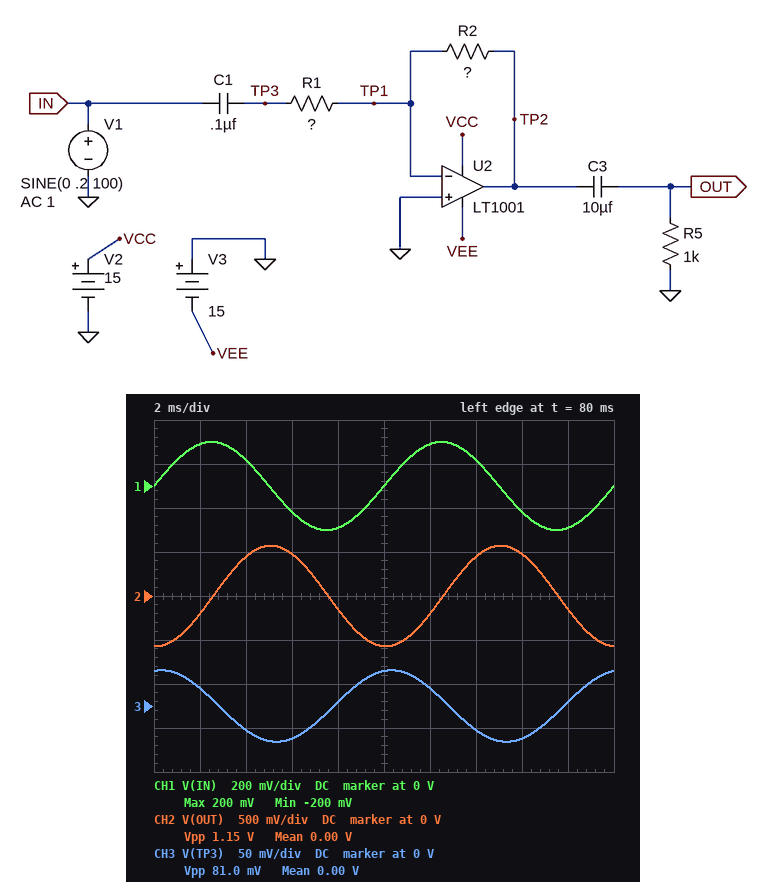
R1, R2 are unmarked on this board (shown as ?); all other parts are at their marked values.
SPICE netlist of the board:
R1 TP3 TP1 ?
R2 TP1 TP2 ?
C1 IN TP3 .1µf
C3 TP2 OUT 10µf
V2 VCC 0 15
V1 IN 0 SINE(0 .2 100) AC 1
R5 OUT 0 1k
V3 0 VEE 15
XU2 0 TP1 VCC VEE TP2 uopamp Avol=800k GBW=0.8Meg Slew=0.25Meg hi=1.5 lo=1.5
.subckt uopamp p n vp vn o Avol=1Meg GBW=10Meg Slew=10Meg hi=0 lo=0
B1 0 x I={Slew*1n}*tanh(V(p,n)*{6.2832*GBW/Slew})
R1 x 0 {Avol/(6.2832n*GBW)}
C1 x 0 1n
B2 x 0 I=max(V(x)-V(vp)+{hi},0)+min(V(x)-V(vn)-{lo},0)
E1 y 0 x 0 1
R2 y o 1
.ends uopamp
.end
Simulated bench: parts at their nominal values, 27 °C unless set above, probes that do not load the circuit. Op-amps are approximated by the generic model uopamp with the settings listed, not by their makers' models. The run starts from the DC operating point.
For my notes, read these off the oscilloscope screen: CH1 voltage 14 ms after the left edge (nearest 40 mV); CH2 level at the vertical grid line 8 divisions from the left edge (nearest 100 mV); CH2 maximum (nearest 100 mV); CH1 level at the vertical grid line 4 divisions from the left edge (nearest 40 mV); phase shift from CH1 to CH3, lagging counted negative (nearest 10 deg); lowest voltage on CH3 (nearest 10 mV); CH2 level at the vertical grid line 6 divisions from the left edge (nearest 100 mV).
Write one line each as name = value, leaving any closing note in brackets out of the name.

CH1 voltage 14 ms after the left edge = 120 mV
CH2 level at the vertical grid line 8 divisions from the left edge = 500 mV
CH2 maximum = 600 mV
CH1 level at the vertical grid line 4 divisions from the left edge = -200 mV
phase shift from CH1 to CH3, lagging counted negative = 80 deg
lowest voltage on CH3 = -40 mV
CH2 level at the vertical grid line 6 divisions from the left edge = -200 mV
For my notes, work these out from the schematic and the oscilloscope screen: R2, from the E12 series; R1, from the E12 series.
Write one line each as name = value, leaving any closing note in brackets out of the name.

R2, from the E12 series = 47 kΩ
R1, from the E12 series = 3.3 kΩ
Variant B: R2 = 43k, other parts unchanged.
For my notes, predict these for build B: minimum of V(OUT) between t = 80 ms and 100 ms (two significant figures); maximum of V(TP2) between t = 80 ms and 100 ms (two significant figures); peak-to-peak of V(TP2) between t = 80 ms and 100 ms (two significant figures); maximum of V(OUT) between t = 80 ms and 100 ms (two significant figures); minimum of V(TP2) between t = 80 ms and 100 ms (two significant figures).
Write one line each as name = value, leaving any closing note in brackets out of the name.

minimum of V(OUT) between t = 80 ms and 100 ms = -520 mV
maximum of V(TP2) between t = 80 ms and 100 ms = 530 mV
peak-to-peak of V(TP2) between t = 80 ms and 100 ms = 1.1 V
maximum of V(OUT) between t = 80 ms and 100 ms = 520 mV
minimum of V(TP2) between t = 80 ms and 100 ms = -530 mV
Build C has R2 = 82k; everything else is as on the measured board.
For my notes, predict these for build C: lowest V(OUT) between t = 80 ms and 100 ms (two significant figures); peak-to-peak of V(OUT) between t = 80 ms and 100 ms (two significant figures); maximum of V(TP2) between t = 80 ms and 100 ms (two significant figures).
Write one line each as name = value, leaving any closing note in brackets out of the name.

lowest V(OUT) between t = 80 ms and 100 ms = -1.0 V
peak-to-peak of V(OUT) between t = 80 ms and 100 ms = 2.0 V
maximum of V(TP2) between t = 80 ms and 100 ms = 1.0 V
